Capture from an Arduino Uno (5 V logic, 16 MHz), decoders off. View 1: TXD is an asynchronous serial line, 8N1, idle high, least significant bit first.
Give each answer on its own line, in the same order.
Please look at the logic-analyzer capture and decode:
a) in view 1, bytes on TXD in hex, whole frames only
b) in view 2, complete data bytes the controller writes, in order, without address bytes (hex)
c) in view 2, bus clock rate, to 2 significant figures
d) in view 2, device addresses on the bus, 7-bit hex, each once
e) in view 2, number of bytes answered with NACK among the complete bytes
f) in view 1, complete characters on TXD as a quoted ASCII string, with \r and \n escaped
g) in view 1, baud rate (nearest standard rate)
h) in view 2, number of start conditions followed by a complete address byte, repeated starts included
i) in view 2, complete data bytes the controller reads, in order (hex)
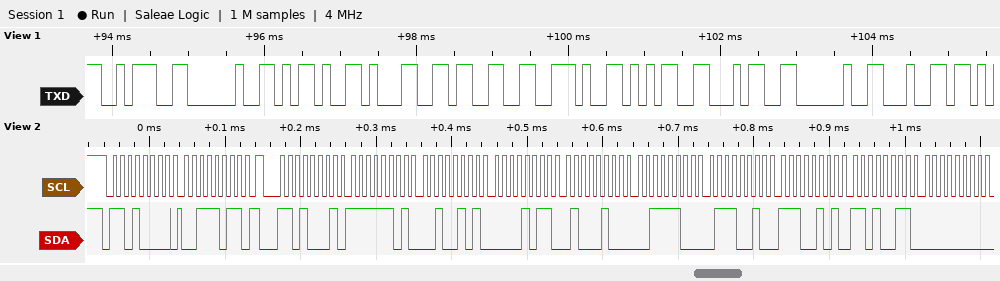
3A 20 2D 31 33 2E 35 34 20 64
3B
100 kHz
0x68
0
": -13.54 d"
9600 baud
2
FD 25 0B 44 3C 72 E5 D3 00
